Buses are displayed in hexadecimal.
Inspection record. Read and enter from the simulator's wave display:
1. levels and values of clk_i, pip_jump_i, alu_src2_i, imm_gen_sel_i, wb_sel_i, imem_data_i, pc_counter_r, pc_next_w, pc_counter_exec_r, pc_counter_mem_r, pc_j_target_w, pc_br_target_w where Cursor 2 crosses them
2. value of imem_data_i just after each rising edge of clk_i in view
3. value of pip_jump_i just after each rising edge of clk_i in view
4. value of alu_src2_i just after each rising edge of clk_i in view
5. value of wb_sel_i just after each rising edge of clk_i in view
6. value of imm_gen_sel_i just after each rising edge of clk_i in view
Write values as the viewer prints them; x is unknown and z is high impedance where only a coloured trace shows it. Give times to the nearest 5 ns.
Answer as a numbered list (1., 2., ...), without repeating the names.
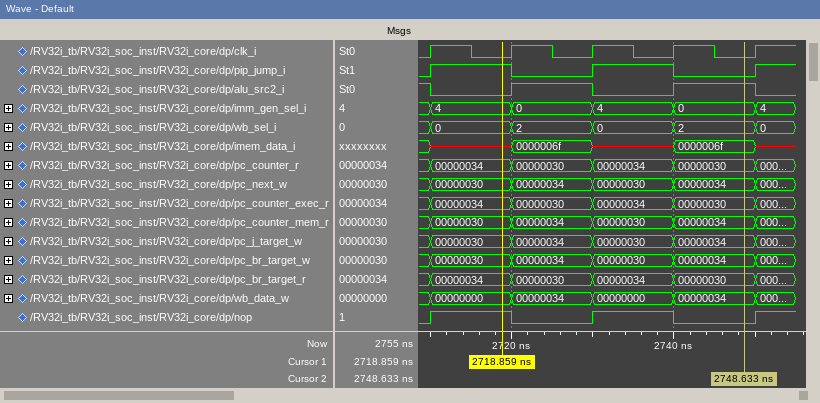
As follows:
1. clk_i=0, pip_jump_i=0, alu_src2_i=1, imm_gen_sel_i=0, wb_sel_i=2, imem_data_i=0000006f, pc_counter_r=00000030, pc_next_w=00000034, pc_counter_exec_r=00000030, pc_counter_mem_r=00000034, pc_j_target_w=00000034, pc_br_target_w=00000034
2. x, 0000006f, x, 0000006f, x
3. 1 0 1 0 1
4. 0 1 0 1 0
5. 0, 2, 0, 2, 0
6. 4, 0, 4, 0, 4
